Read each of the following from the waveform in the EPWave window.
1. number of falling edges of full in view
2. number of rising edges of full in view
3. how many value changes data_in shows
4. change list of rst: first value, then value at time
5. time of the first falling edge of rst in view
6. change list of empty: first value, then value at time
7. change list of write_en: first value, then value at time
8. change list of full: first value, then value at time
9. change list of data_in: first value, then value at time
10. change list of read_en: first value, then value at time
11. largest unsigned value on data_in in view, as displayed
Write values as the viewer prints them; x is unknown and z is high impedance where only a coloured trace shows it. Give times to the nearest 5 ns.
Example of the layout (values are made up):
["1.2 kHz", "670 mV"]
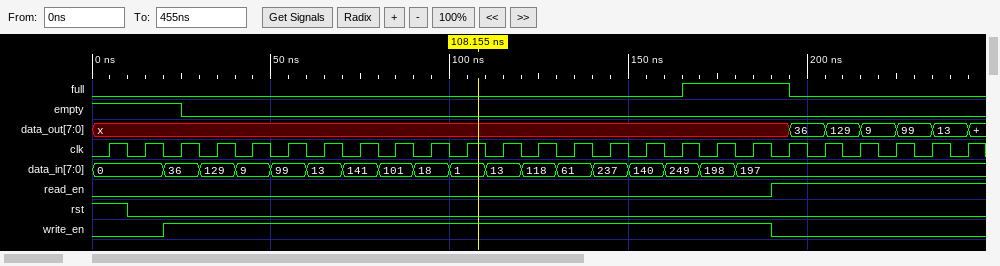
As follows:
["1", "1", "17", "1, 0 at 10 ns", "10 ns", "1, 0 at 25 ns", "0, 1 at 20 ns, 0 at 190 ns", "0, 1 at 165 ns, 0 at 195 ns", "0, 36 at 20 ns, 129 at 30 ns, 9 at 40 ns, 99 at 50 ns, 13 at 60 ns, 141 at 70 ns, 101 at 80 ns, 18 at 90 ns, 1 at 100 ns, 13 at 110 ns, 118 at 120 ns, 61 at 130 ns, 237 at 140 ns, 140 at 150 ns, 249 at 160 ns, 198 at 170 ns, 197 at 180 ns", "0, 1 at 190 ns", "249"]
